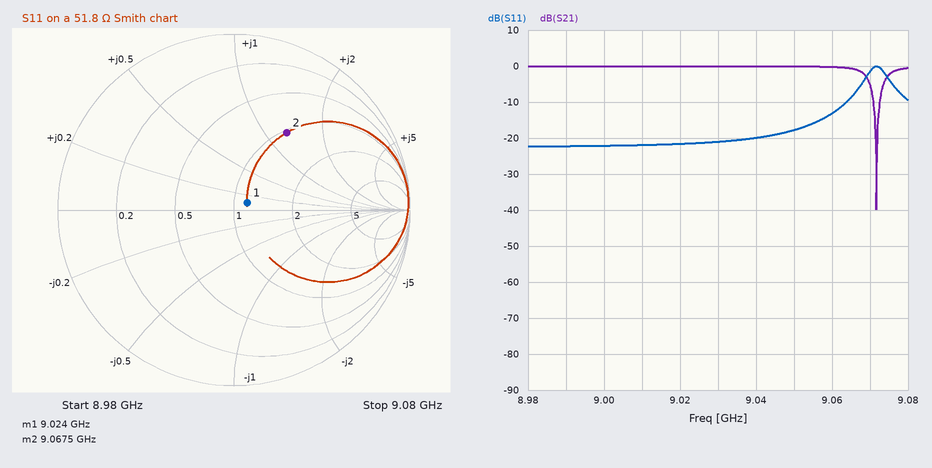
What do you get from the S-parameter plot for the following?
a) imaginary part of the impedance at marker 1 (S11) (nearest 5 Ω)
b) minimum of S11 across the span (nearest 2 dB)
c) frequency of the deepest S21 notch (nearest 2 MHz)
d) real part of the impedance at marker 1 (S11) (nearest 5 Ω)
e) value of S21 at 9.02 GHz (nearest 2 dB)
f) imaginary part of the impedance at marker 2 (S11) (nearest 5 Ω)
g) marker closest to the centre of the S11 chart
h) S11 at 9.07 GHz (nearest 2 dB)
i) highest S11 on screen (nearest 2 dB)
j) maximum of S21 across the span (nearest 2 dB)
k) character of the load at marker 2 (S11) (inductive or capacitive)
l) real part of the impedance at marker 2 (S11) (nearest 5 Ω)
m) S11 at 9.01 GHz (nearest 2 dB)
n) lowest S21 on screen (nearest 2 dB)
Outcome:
+5 Ω
-22 dB
9.072 GHz
60 Ω
0 dB
+65 Ω
marker 1
-2 dB
0 dB
0 dB
inductive
55 Ω
-22 dB
-40 dB
